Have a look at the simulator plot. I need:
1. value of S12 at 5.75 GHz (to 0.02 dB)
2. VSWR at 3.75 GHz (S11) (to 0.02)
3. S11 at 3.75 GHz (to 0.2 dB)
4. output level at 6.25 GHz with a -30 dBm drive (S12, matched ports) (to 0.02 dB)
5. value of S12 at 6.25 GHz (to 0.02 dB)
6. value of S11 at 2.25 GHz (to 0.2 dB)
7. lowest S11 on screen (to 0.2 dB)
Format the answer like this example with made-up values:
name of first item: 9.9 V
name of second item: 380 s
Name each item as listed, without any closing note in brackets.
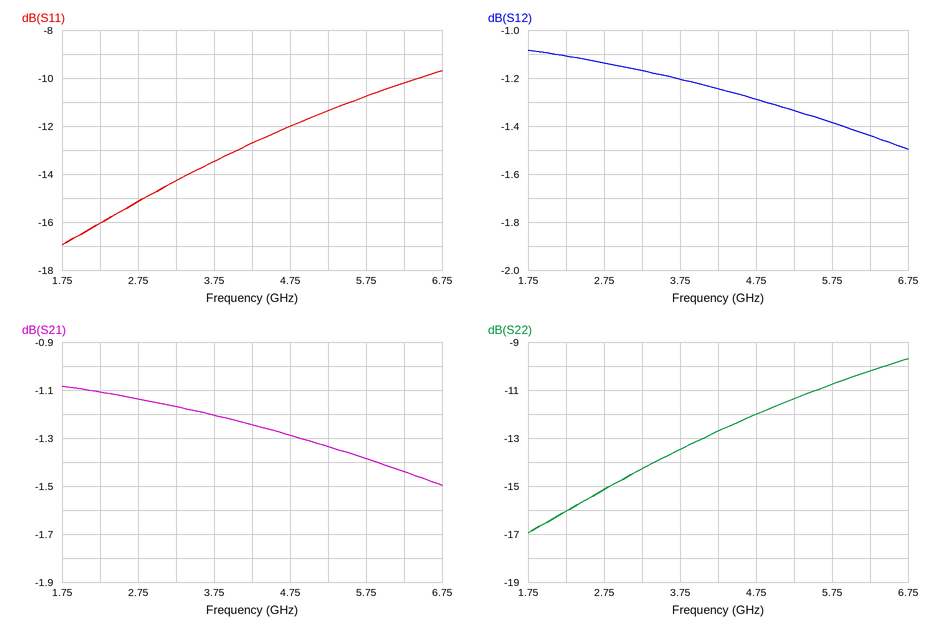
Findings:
value of S12 at 5.75 GHz: -1.38 dB
VSWR at 3.75 GHz (S11): 1.54
S11 at 3.75 GHz: -13.4 dB
output level at 6.25 GHz with a -30 dBm drive (S12, matched ports): -31.44 dBm
value of S12 at 6.25 GHz: -1.44 dB
value of S11 at 2.25 GHz: -16.0 dB
lowest S11 on screen: -17.0 dB
